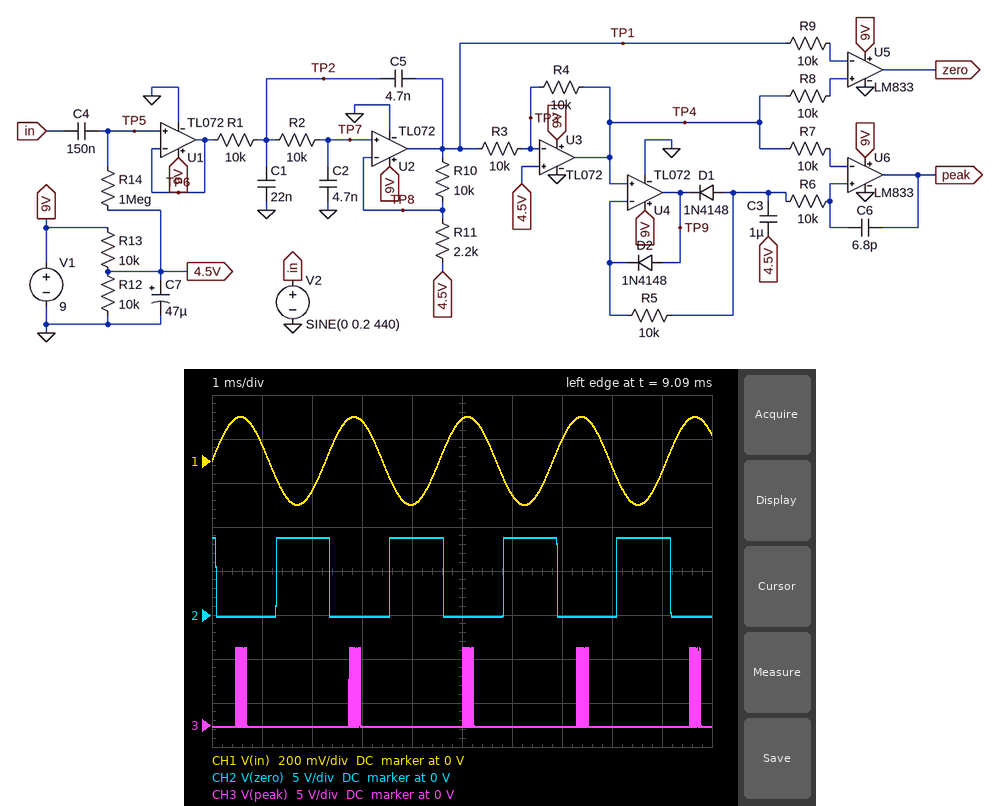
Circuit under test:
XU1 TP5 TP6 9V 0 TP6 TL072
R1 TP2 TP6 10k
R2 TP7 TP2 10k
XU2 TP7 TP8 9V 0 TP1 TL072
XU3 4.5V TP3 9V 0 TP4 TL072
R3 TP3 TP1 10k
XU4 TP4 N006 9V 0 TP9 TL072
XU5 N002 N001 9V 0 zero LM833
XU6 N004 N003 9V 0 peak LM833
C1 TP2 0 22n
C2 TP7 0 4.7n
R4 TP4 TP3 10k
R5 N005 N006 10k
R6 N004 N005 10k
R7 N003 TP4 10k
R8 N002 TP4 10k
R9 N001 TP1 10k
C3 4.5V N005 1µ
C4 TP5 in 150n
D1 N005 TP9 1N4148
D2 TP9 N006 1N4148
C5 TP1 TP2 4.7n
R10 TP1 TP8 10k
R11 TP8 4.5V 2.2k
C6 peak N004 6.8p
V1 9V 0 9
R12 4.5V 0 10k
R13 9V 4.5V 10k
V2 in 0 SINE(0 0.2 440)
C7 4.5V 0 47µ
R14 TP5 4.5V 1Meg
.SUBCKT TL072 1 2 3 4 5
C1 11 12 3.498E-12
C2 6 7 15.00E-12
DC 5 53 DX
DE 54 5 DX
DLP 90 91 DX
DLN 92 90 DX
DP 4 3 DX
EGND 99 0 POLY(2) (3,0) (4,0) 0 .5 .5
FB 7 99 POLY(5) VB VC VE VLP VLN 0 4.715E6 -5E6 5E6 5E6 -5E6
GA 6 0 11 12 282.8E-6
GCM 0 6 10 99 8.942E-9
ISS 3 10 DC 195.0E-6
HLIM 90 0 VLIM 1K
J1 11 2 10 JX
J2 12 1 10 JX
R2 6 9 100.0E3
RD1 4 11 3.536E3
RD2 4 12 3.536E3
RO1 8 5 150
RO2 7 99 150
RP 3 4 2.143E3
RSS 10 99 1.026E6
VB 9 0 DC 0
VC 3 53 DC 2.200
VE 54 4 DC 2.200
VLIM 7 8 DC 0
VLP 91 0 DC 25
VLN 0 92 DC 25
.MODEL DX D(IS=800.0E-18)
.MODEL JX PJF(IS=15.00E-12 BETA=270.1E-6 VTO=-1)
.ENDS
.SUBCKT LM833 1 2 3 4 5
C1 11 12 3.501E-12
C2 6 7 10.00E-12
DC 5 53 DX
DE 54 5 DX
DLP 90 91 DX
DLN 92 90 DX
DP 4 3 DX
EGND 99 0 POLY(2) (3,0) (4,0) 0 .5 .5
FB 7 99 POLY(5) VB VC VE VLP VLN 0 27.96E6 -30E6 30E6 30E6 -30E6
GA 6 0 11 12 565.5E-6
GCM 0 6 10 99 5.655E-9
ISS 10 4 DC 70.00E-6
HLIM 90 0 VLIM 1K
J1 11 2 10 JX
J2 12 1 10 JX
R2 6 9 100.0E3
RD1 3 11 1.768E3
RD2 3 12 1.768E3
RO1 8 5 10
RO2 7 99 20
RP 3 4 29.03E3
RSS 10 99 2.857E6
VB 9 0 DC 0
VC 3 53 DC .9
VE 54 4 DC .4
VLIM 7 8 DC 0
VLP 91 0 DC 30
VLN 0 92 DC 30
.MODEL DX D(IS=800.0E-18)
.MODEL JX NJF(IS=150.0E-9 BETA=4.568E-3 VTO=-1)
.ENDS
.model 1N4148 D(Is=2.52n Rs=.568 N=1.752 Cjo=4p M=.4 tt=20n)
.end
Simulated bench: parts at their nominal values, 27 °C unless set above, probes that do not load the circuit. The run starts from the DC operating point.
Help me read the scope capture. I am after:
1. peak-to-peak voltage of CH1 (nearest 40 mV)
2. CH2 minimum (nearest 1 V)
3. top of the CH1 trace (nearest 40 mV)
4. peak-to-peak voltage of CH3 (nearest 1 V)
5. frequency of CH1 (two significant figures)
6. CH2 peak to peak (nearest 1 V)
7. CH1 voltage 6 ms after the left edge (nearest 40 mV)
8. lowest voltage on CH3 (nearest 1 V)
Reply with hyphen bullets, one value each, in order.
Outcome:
- 400 mV
- 0 V
- 200 mV
- 9 V
- 440 Hz
- 9 V
- -160 mV
- 0 V
